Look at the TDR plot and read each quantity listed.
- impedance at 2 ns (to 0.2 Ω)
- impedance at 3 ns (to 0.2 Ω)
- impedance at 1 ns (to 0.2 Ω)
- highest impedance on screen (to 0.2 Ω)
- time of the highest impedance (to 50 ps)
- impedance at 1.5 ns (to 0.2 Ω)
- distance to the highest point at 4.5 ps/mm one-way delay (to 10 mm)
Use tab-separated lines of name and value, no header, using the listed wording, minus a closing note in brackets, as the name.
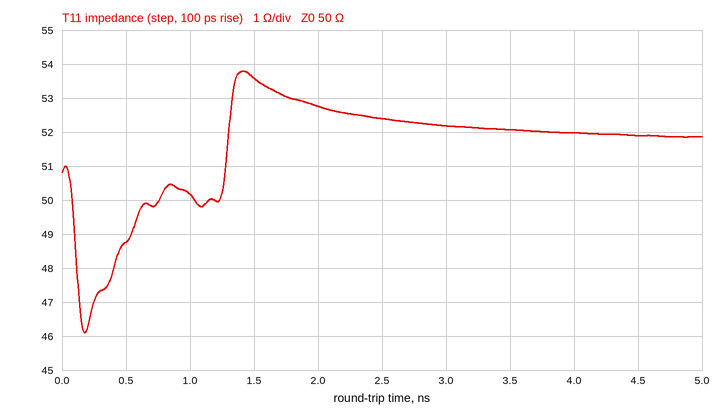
impedance at 2 ns	52.8 Ω
impedance at 3 ns	52.2 Ω
impedance at 1 ns	50.2 Ω
highest impedance on screen	53.8 Ω
time of the highest impedance	1.40 ns
impedance at 1.5 ns	53.6 Ω
distance to the highest point at 4.5 ps/mm one-way delay	160 mm
